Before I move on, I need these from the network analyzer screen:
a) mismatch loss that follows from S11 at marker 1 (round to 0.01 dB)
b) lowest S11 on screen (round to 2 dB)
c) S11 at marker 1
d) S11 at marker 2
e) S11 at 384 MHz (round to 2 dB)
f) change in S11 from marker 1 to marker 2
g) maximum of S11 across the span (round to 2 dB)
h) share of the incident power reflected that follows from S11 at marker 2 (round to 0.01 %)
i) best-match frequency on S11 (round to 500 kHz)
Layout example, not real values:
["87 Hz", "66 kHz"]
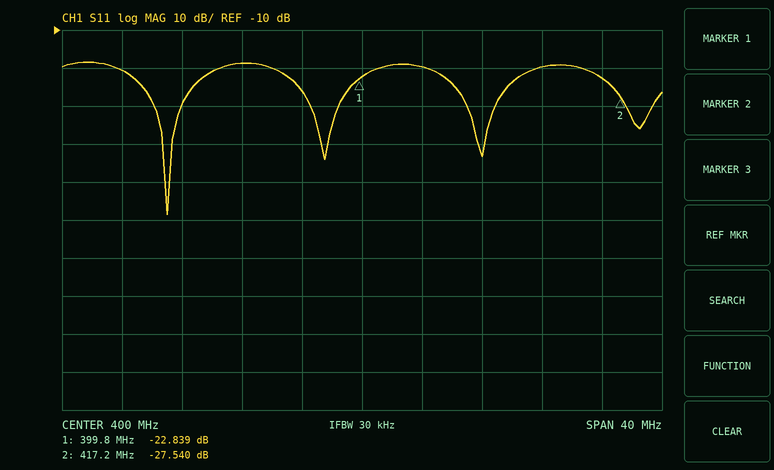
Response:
["0.02 dB", "-58 dB", "-22.839 dB", "-27.540 dB", "-20 dB", "-4.701 dB", "-18 dB", "0.18 %", "387.0 MHz"]
